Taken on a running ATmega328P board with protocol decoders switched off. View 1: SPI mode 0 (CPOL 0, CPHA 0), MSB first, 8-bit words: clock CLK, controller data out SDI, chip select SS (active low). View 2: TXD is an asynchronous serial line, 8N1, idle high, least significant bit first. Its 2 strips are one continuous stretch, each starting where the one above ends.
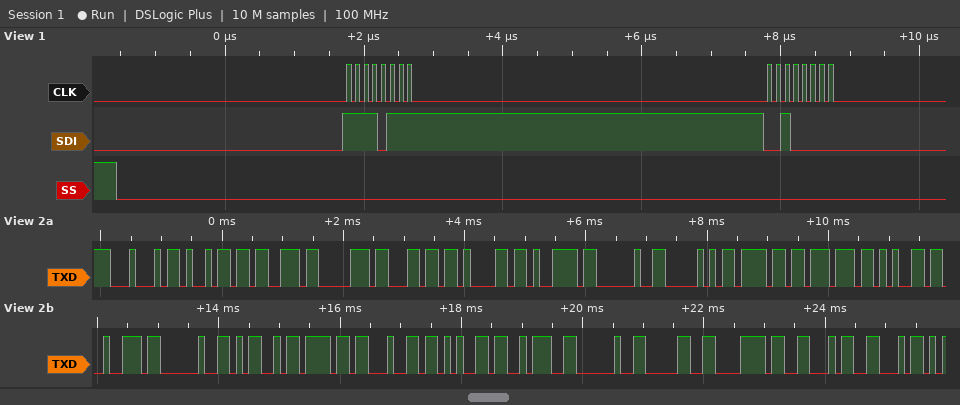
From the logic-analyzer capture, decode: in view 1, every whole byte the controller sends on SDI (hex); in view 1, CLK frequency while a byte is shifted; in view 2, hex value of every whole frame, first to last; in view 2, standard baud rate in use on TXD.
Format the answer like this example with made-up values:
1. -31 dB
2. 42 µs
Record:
1. F7 20
2. 8 MHz
3. 0x44 0x69 0x73 0x70 0x6C 0x61 0x79 0x20 0x50 0x6F 0x77 0x65 0x72 0x20 0x4D 0x6F 0x64 0x65 0x3A 0x20 0x30 0x78 0x46 0x46
4. 9600 baud
